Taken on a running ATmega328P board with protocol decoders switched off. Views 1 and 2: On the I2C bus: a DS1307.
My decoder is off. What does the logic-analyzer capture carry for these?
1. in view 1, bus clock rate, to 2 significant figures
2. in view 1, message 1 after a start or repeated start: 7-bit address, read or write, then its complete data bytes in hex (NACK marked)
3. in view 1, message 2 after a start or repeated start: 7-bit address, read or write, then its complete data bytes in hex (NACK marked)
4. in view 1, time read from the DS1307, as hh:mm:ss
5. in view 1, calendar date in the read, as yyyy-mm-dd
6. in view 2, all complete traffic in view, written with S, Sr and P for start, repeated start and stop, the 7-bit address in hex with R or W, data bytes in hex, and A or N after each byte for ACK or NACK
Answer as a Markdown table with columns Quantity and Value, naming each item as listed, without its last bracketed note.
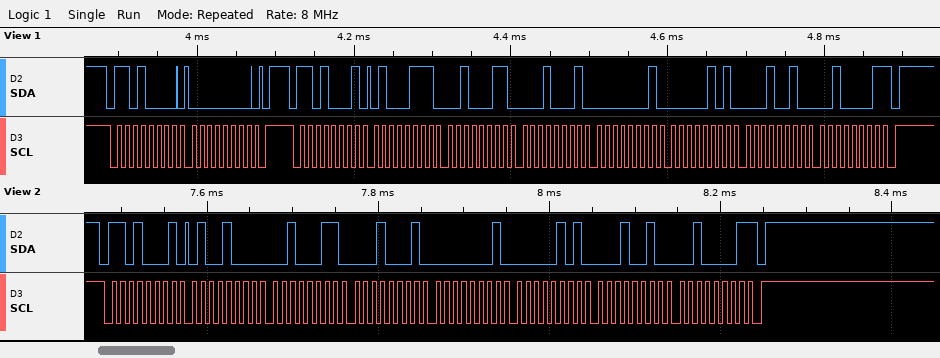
| Quantity | Value |
|---|---|
| in view 1, bus clock rate, to 2 significant figures | 100 kHz |
| in view 1, message 1 after a start or repeated start: 7-bit address, read or write, then its complete data bytes in hex | 0x68 write: 00 |
| in view 1, message 2 after a start or repeated start: 7-bit address, read or write, then its complete data bytes in hex | 0x68 read: 47 23 11 01 05 12 21 NACK |
| in view 1, time read from the DS1307, as hh:mm:ss | 11:23:47 |
| in view 1, calendar date in the read, as yyyy-mm-dd | 2021-12-05 |
| in view 2, all complete traffic in view, written with S, Sr and P for start, repeated start and stop, the 7-bit address in hex with R or W, data bytes in hex, and A or N after each byte for ACK or NACK | S 68R A 48 A 23 A 11 A 01 A 05 A 12 A 21 N P |
